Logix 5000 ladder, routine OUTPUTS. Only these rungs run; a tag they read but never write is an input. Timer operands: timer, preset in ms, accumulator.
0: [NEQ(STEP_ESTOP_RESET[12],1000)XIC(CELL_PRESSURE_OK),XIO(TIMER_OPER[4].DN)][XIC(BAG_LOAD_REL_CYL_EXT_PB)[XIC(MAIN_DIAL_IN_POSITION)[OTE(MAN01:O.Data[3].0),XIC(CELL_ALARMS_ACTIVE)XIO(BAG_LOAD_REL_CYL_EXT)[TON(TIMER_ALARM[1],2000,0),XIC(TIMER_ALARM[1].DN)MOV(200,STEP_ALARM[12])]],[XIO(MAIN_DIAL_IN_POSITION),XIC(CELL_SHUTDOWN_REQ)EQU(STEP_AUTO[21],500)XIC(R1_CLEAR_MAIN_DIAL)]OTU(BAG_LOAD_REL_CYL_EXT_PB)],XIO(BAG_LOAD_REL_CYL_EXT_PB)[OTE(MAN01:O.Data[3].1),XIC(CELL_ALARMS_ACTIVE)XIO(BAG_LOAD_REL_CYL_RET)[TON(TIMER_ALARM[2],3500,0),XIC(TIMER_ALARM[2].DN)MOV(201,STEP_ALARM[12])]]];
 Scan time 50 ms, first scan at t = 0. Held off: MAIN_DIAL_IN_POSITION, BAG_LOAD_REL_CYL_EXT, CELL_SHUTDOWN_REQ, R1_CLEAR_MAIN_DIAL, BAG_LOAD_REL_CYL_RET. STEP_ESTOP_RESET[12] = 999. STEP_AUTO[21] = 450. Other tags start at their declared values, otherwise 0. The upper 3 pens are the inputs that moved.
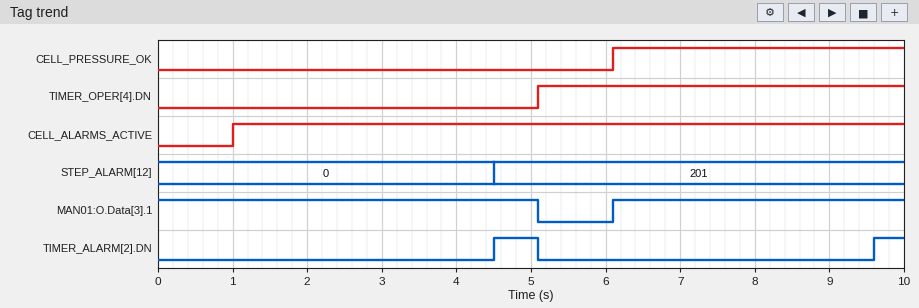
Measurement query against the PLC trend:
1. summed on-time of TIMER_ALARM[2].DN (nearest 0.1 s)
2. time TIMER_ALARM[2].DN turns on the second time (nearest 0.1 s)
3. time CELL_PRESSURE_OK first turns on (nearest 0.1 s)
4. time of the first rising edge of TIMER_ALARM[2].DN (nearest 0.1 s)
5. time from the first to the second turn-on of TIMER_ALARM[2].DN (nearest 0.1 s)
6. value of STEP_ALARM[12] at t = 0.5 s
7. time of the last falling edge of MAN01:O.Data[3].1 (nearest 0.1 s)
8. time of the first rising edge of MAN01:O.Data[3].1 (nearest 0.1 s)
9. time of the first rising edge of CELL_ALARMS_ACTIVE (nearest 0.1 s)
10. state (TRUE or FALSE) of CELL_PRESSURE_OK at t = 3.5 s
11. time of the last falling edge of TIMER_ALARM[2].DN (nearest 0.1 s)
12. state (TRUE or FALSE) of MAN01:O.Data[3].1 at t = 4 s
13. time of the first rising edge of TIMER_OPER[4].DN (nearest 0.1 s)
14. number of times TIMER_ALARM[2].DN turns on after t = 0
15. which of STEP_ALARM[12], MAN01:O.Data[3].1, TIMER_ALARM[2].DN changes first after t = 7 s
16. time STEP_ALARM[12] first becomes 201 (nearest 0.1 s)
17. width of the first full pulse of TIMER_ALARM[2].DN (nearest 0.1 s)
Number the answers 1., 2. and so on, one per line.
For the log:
1. 1.0 s
2. 9.6 s
3. 6.1 s
4. 4.5 s
5. 5.1 s
6. 0
7. 5.1 s
8. 6.1 s
9. 1.0 s
10. FALSE
11. 5.1 s
12. TRUE
13. 5.1 s
14. 2
15. TIMER_ALARM[2].DN
16. 4.5 s
17. 0.6 s
